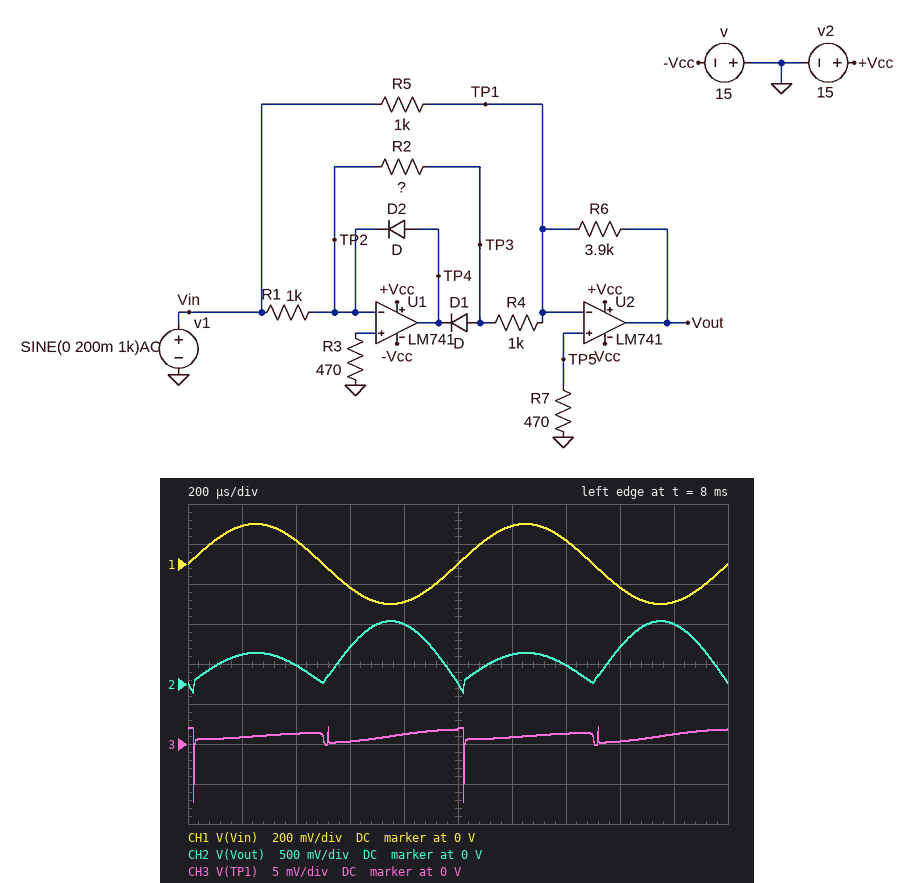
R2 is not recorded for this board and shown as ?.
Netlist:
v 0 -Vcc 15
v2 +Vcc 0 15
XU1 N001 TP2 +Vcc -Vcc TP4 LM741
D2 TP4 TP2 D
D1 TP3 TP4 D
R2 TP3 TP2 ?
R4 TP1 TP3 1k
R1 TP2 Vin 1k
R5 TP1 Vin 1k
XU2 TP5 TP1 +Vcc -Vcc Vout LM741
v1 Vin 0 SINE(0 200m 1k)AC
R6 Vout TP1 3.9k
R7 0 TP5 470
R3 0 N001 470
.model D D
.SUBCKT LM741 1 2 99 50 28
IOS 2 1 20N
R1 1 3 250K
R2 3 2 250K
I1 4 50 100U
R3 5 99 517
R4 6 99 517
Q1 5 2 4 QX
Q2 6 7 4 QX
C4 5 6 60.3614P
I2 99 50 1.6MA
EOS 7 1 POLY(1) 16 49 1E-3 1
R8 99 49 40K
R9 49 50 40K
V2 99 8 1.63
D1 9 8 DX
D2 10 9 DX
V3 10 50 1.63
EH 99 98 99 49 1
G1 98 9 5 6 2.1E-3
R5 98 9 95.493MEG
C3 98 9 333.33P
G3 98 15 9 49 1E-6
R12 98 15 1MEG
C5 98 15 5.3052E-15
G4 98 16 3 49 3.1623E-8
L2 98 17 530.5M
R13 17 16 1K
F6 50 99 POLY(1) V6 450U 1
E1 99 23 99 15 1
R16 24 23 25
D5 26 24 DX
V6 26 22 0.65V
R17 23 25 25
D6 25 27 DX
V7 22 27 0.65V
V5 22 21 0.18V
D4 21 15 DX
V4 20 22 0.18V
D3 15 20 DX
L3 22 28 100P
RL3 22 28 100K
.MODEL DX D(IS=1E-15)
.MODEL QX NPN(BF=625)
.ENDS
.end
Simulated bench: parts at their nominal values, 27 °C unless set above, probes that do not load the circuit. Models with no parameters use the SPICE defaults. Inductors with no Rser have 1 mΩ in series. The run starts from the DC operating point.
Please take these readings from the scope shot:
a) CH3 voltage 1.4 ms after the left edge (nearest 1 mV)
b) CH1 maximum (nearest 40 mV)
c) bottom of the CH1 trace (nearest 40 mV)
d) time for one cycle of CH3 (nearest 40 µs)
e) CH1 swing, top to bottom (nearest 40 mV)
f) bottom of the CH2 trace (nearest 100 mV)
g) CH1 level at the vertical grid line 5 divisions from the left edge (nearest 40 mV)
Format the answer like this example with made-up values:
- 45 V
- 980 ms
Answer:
- 1 mV
- 200 mV
- -200 mV
- 1.00 ms
- 400 mV
- -100 mV
- 0 V
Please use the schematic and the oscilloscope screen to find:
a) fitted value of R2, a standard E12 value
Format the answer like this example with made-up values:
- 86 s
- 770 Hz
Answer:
- 1.5 kΩ
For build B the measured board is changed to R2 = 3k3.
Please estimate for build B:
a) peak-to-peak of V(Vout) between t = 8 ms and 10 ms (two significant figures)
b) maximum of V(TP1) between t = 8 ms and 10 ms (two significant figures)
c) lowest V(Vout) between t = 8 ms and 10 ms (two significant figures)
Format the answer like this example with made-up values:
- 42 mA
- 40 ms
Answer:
- 1.9 V
- 2.8 mV
- -94 mV
